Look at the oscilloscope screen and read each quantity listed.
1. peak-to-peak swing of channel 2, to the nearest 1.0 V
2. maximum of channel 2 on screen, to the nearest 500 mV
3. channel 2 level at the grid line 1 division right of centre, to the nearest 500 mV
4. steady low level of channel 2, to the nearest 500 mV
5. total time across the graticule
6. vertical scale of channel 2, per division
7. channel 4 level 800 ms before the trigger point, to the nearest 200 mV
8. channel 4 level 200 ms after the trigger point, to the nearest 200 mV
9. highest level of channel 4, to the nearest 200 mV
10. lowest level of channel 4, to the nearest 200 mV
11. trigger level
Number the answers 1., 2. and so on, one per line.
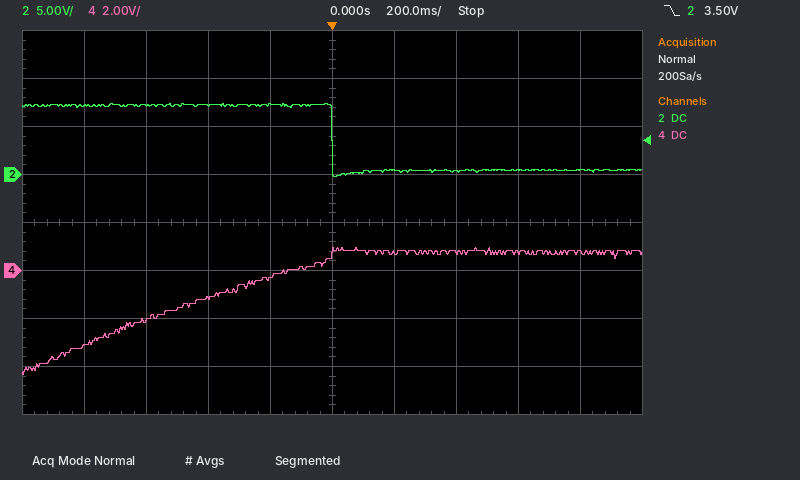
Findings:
1. 8.0 V
2. 7.5 V
3. 500 mV
4. 500 mV
5. 2 s
6. 5 V
7. -3.2 V
8. 800 mV
9. 1.0 V
10. -4.4 V
11. 3.50 V
